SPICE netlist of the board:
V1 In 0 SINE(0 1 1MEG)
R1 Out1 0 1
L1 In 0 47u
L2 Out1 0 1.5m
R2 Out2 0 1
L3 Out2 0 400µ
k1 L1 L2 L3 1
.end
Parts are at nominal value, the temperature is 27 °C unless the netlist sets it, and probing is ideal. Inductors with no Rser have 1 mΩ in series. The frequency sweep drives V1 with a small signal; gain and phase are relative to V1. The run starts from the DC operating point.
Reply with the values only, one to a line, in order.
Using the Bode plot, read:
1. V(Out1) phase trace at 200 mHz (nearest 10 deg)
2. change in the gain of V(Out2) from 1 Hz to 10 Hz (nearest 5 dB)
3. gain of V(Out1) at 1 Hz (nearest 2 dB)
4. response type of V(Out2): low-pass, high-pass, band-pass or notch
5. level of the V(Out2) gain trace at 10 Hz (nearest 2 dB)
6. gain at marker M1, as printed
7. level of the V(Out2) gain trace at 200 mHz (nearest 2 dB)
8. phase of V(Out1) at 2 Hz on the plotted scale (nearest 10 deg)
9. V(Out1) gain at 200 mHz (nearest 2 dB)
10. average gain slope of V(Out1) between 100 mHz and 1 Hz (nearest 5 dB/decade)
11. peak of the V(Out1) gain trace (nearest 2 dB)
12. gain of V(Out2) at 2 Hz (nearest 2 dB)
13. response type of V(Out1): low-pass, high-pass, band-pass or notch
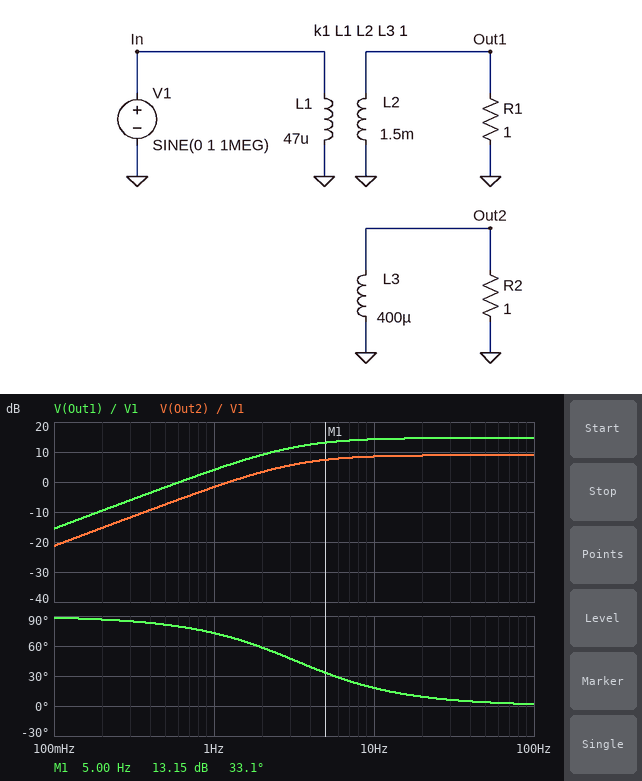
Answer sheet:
90 deg
10 dB
4 dB
high-pass
8 dB
13.15 dB
-16 dB
60 deg
-10 dB
20 dB/decade
14 dB
4 dB
high-pass
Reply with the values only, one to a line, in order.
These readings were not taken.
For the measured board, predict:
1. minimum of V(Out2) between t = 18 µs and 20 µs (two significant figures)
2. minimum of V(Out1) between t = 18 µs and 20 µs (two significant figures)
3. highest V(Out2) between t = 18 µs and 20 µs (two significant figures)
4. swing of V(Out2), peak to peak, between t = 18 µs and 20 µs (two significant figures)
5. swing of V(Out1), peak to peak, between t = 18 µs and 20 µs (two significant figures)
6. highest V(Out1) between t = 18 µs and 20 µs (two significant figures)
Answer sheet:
-2.8 V
-5.4 V
2.8 V
5.6 V
11 V
5.4 V
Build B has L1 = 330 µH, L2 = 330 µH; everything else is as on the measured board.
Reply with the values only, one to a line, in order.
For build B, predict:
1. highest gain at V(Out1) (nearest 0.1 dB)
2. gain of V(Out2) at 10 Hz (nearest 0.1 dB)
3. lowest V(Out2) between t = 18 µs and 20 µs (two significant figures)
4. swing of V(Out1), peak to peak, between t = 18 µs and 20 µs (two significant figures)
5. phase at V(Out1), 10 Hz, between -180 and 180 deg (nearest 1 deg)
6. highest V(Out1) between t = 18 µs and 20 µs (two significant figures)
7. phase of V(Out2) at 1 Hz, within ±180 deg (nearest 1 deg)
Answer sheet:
0 dB
0.8 dB
-1.1 V
2.0 V
3 deg
1.0 V
26 deg
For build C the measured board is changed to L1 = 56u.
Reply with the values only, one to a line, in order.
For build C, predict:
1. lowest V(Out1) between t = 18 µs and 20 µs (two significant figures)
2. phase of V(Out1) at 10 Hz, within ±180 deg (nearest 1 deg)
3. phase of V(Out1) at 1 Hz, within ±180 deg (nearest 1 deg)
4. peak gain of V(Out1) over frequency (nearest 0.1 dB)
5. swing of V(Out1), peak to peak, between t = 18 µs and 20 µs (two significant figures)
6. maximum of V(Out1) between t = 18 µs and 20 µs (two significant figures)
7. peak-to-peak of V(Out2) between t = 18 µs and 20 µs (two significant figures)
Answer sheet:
-5.0 V
15 deg
70 deg
14.0 dB
10 V
5.0 V
5.2 V
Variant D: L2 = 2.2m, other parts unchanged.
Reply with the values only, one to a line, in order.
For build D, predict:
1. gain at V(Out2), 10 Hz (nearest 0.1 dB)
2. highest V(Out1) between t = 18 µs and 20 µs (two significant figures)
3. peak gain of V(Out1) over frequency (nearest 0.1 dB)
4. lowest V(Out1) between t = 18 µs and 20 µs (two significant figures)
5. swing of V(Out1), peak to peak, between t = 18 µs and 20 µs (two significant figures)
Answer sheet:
8.4 dB
6.5 V
16.2 dB
-6.5 V
13 V
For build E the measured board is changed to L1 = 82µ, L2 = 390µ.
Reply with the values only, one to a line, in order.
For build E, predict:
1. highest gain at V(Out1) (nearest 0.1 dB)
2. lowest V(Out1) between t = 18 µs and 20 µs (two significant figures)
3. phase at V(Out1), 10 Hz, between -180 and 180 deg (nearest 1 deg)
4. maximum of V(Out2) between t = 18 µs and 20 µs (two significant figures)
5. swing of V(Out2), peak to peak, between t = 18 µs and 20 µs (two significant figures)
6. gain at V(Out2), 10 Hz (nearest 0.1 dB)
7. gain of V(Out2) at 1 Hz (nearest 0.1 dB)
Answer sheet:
6.7 dB
-2.2 V
11 deg
2.2 V
4.4 V
6.6 dB
0.1 dB
